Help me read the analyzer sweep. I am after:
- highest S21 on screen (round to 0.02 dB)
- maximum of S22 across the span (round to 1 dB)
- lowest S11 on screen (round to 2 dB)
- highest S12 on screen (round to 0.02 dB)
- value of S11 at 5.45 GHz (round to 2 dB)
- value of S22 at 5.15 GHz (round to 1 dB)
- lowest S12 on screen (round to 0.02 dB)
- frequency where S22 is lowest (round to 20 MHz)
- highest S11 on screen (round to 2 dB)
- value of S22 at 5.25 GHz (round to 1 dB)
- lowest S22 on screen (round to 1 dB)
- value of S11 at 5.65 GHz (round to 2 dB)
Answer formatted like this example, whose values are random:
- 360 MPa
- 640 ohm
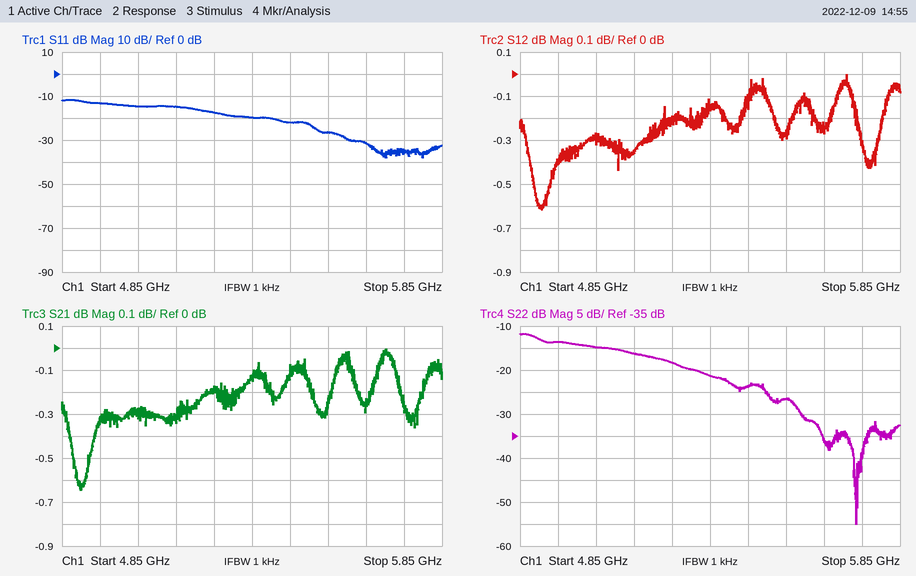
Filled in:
- 0.00 dB
- -12 dB
- -38 dB
- 0.00 dB
- -22 dB
- -16 dB
- -0.62 dB
- 5.74 GHz
- -12 dB
- -18 dB
- -55 dB
- -32 dB
